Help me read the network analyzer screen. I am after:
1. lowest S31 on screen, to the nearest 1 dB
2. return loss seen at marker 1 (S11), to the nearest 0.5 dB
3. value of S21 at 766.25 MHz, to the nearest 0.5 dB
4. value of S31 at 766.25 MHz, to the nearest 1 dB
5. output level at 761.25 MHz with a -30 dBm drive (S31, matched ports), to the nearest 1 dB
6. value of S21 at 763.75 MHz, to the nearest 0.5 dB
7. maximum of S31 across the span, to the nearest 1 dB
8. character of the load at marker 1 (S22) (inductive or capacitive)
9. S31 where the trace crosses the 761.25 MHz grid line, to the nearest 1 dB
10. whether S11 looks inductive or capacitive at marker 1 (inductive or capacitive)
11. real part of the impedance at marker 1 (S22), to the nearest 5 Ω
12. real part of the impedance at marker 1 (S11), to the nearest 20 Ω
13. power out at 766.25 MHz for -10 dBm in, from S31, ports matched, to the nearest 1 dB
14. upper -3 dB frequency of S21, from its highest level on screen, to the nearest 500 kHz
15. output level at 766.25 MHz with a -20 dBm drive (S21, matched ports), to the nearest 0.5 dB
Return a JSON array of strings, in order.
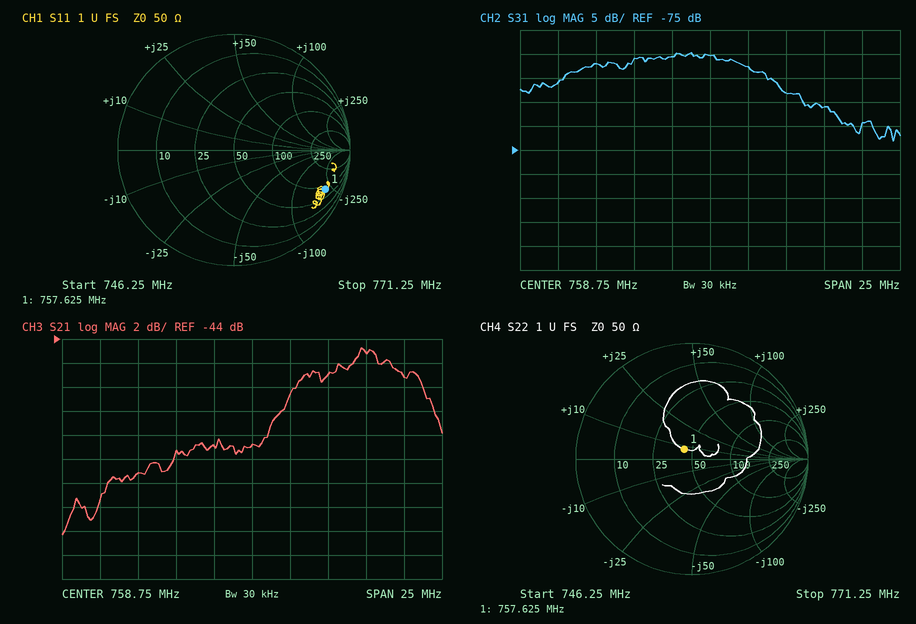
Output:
["-73 dB", "1.5 dB", "-45.0 dB", "-66 dB", "-88 dBm", "-47.0 dB", "-55 dB", "inductive", "-58 dB", "capacitive", "45 Ω", "80 Ω", "-76 dBm", "770.0 MHz", "-65.0 dBm"]
